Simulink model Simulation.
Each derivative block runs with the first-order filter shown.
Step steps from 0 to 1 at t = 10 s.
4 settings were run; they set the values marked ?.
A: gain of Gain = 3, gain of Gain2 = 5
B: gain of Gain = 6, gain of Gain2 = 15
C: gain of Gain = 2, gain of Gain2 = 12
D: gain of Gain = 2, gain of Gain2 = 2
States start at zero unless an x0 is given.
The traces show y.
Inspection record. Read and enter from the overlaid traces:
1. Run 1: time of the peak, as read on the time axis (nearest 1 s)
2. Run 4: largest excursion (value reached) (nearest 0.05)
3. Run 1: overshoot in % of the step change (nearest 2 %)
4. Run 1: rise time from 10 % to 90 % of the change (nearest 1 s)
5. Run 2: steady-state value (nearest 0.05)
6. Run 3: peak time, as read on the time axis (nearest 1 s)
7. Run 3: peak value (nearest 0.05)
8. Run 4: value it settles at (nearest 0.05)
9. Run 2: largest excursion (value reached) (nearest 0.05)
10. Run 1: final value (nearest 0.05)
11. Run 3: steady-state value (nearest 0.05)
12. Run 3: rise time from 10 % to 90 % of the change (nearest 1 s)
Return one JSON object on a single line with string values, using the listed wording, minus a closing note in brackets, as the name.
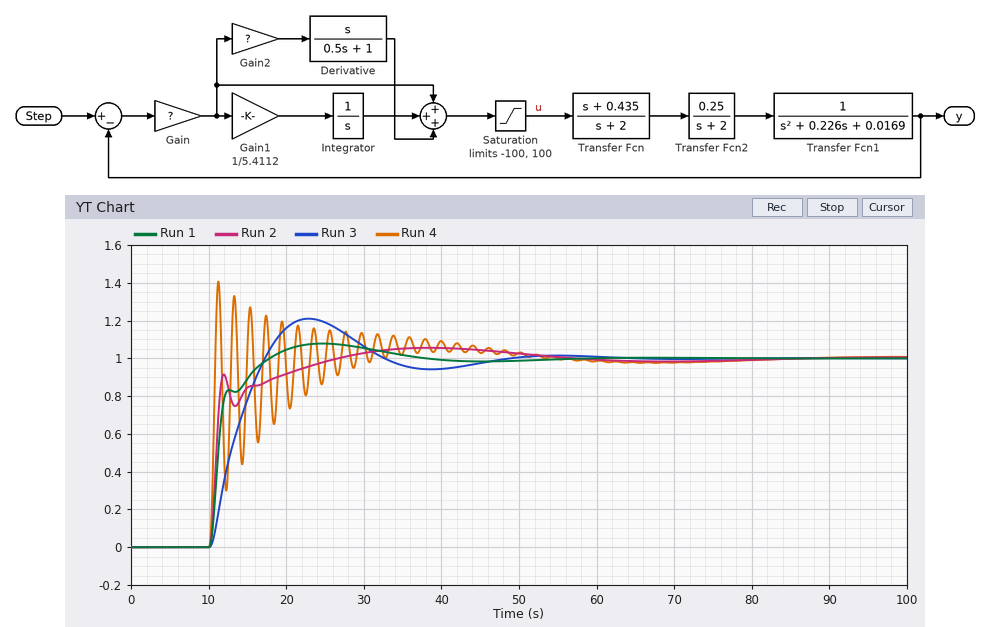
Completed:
{"Run 1: time of the peak, as read on the time axis": "25 s", "Run 4: largest excursion (value reached)": "1.40", "Run 1: overshoot in % of the step change": "8 %", "Run 1: rise time from 10 % to 90 % of the change": "5 s", "Run 2: steady-state value": "1.00", "Run 3: peak time, as read on the time axis": "23 s", "Run 3: peak value": "1.20", "Run 4: value it settles at": "1.00", "Run 2: largest excursion (value reached)": "1.05", "Run 1: final value": "1.00", "Run 3: steady-state value": "1.00", "Run 3: rise time from 10 % to 90 % of the change": "5 s"}
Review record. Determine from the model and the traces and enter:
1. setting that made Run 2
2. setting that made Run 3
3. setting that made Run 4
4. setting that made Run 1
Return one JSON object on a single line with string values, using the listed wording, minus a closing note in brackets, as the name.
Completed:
{"setting that made Run 2": "C", "setting that made Run 3": "D", "setting that made Run 4": "B", "setting that made Run 1": "A"}
